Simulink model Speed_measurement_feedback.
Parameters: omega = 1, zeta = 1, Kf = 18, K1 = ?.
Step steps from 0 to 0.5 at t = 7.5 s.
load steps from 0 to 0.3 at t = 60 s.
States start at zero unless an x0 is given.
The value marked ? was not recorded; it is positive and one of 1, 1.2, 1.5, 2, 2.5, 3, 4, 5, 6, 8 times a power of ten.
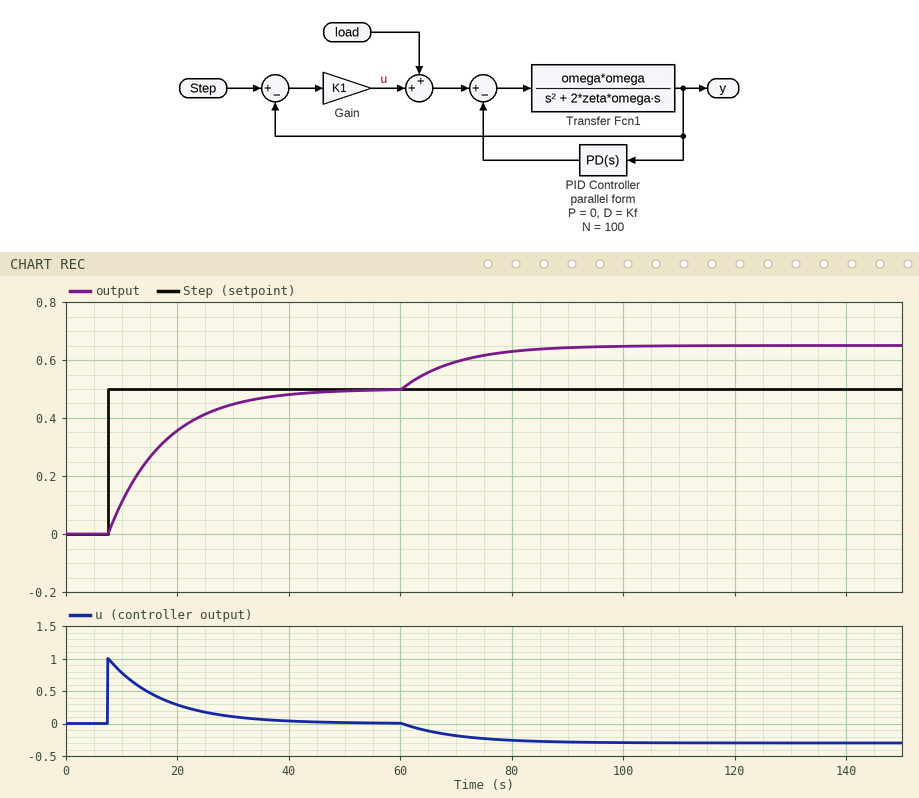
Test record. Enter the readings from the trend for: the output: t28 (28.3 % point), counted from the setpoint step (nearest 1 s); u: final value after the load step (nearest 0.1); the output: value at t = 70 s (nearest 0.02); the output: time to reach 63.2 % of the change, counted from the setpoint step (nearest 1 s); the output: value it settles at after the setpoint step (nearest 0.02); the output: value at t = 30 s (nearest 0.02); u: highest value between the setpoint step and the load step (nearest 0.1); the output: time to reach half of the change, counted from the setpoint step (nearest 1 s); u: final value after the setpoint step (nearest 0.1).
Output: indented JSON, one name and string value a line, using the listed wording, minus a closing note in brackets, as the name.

{
  "the output: t28 (28.3 % point), counted from the setpoint step": "3 s",
  "u: final value after the load step": "-0.3",
  "the output: value at t = 70 s": "0.60",
  "the output: time to reach 63.2 % of the change, counted from the setpoint step": "10 s",
  "the output: value it settles at after the setpoint step": "0.50",
  "the output: value at t = 30 s": "0.44",
  "u: highest value between the setpoint step and the load step": "1.0",
  "the output: time to reach half of the change, counted from the setpoint step": "7 s",
  "u: final value after the setpoint step": "0.0"
}
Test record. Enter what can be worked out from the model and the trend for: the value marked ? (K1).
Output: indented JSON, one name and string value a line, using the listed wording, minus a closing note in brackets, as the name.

{
  "the value marked ?": "2"
}
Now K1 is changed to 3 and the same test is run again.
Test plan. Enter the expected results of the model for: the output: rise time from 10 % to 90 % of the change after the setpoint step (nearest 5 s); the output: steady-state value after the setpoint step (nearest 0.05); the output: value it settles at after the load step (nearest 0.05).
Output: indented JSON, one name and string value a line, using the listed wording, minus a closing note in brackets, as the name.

{
  "the output: rise time from 10 % to 90 % of the change after the setpoint step": "15 s",
  "the output: steady-state value after the setpoint step": "0.50",
  "the output: value it settles at after the load step": "0.60"
}
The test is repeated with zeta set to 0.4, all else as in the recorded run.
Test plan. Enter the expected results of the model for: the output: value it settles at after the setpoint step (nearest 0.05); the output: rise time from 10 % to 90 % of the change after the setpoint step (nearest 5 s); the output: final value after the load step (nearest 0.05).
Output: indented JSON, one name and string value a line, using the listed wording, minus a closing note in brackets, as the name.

{
  "the output: value it settles at after the setpoint step": "0.50",
  "the output: rise time from 10 % to 90 % of the change after the setpoint step": "20 s",
  "the output: final value after the load step": "0.65"
}
